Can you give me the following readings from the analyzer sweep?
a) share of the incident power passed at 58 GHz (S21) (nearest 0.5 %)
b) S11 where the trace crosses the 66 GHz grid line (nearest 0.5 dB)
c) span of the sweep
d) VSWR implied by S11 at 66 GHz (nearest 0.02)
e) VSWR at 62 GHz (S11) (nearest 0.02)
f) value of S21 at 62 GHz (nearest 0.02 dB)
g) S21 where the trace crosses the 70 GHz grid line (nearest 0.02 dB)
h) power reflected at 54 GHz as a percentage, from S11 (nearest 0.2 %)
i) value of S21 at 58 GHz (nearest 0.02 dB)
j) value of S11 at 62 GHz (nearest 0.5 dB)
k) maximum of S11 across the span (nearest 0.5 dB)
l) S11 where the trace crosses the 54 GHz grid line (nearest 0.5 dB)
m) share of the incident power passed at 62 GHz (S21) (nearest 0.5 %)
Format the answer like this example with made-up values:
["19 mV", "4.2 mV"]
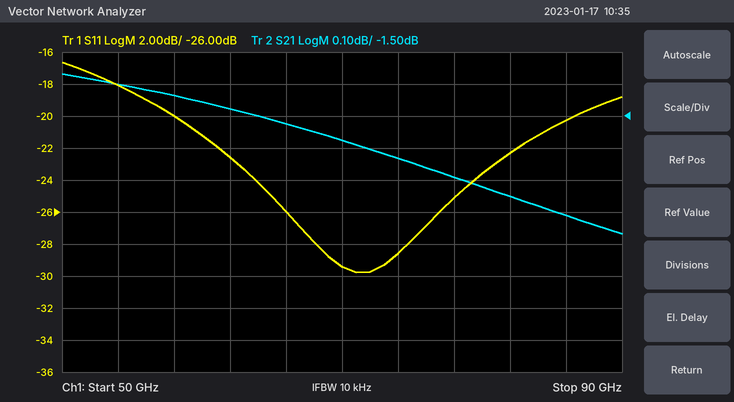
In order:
["72.0 %", "-26.0 dB", "40 GHz", "1.10", "1.16", "-1.48 dB", "-1.58 dB", "1.6 %", "-1.44 dB", "-22.5 dB", "-16.5 dB", "-18.0 dB", "71.0 %"]
